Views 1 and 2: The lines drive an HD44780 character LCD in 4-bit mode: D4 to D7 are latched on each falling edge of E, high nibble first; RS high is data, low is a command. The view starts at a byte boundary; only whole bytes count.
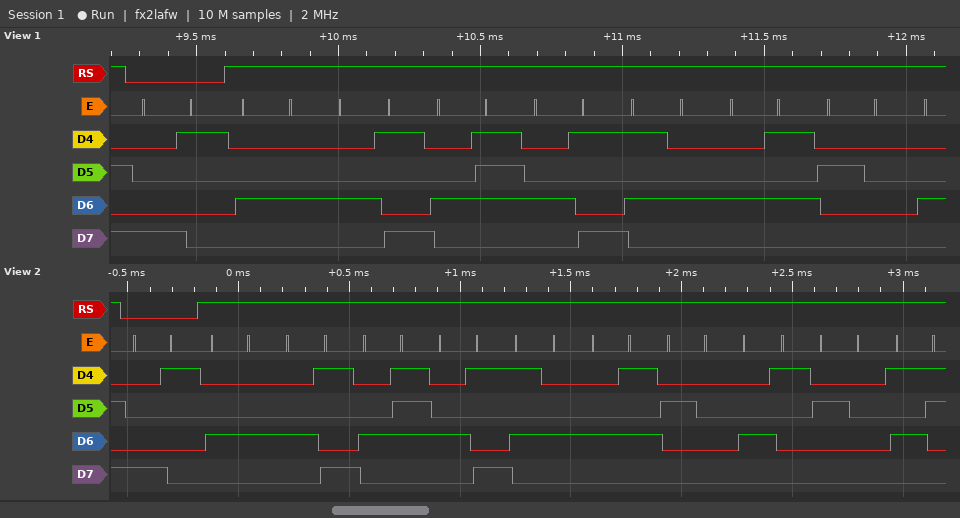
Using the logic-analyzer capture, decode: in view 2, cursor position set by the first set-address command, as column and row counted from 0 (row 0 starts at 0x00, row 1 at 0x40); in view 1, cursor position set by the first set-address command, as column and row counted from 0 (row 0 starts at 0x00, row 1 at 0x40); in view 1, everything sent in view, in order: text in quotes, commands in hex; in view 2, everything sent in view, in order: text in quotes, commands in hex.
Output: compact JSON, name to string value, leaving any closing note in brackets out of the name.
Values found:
{"in view 2, cursor position set by the first set-address command, as column and row counted from 0": "column 1, row 0", "in view 1, cursor position set by the first set-address command, as column and row counted from 0": "column 1, row 0", "in view 1, everything sent in view, in order: text in quotes, commands in hex": "0x81 \"DIGITE \"", "in view 2, everything sent in view, in order: text in quotes, commands in hex": "0x81 \"DIGITE A S\""}
